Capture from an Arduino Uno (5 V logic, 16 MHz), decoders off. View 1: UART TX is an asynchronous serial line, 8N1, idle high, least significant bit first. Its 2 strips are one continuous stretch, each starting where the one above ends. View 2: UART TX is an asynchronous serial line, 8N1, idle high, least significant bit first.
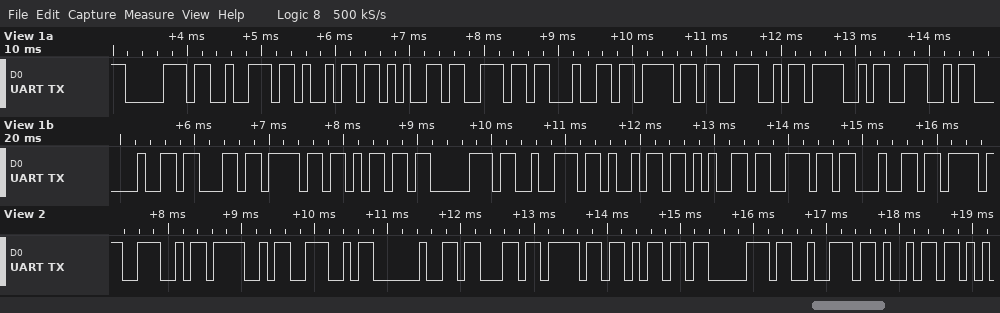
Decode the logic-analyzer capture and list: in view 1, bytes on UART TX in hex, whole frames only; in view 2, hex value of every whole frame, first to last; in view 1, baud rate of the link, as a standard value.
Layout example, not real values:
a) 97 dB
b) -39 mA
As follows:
a) 70 72 69 65 6E 64 6F 4E 4F 4E 20 63 6F 6D 70 72 69 65 6E 64
b) 4E 4F 4E 20 63 6F 6D 70 72 69
c) 9600 baud
